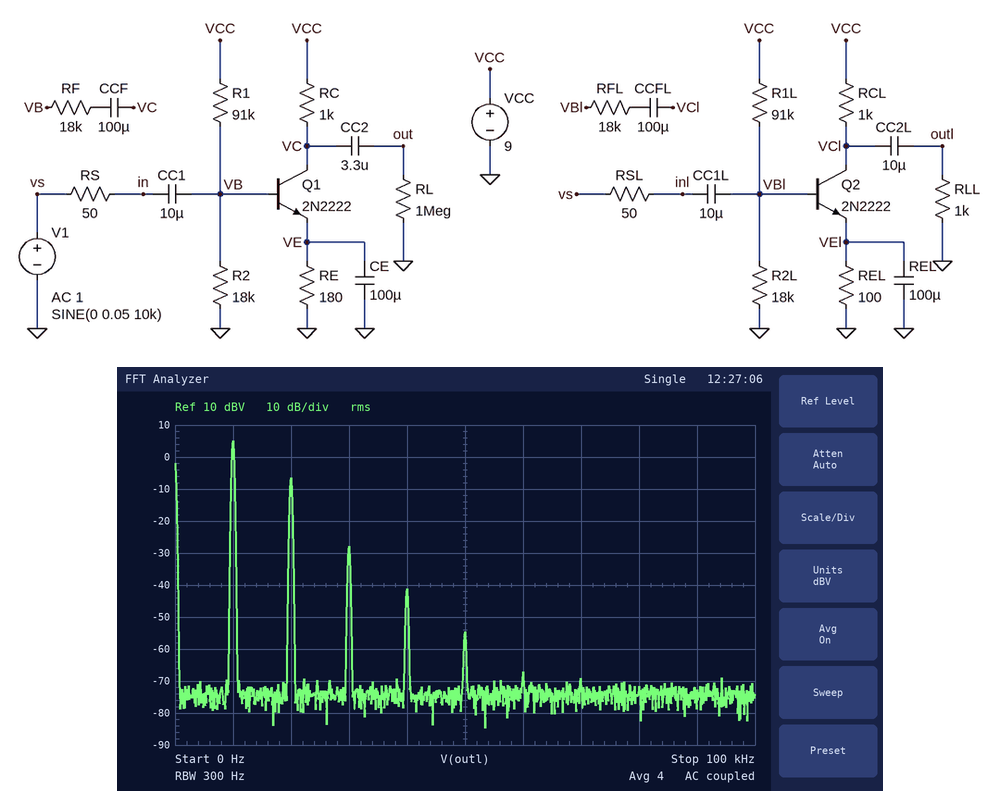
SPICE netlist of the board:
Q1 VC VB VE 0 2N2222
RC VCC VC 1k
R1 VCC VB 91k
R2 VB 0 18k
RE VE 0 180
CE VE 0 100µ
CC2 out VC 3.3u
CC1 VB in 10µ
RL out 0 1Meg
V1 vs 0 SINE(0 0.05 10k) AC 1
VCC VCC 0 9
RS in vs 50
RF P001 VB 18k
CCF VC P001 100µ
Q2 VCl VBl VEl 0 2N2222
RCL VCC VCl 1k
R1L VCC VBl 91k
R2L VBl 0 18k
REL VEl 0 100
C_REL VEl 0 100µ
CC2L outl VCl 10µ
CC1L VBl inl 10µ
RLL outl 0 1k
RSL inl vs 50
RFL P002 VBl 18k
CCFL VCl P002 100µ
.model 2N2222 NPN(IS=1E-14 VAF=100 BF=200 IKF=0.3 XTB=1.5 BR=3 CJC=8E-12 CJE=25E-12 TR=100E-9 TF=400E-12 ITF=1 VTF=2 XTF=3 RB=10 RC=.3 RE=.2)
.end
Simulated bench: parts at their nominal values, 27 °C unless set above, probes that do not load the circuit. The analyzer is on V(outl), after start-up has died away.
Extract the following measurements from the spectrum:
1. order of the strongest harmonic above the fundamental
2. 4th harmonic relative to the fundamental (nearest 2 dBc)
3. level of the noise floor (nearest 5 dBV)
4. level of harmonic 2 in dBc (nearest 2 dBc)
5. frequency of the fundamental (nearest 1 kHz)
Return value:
2
-46 dBc
-75 dBV
-12 dBc
10 kHz
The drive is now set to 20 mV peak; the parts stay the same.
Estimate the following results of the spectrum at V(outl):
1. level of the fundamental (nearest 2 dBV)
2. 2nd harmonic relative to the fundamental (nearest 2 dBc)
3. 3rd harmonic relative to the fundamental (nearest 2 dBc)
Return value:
-2 dBV
-20 dBc
-54 dBc
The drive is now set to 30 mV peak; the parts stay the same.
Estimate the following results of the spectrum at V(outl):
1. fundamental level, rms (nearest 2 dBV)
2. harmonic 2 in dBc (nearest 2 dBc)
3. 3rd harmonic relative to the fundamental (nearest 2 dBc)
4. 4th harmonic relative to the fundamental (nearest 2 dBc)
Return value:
2 dBV
-16 dBc
-44 dBc
-58 dBc
